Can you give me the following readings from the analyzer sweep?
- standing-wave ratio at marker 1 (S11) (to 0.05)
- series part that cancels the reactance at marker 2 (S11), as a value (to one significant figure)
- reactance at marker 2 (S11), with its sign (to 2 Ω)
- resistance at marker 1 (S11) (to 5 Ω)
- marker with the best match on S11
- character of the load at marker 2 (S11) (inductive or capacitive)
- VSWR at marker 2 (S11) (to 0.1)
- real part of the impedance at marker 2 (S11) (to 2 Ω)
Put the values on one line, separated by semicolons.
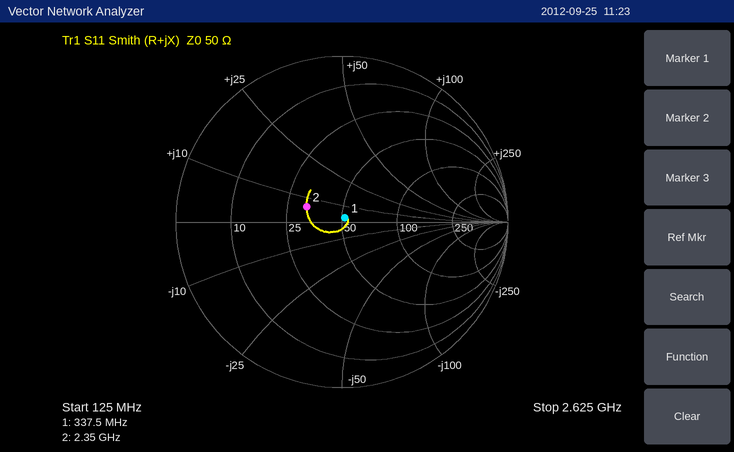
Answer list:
1.05; 10 pF; +6 Ω; 50 Ω; marker 1; inductive; 1.6; 32 Ω
